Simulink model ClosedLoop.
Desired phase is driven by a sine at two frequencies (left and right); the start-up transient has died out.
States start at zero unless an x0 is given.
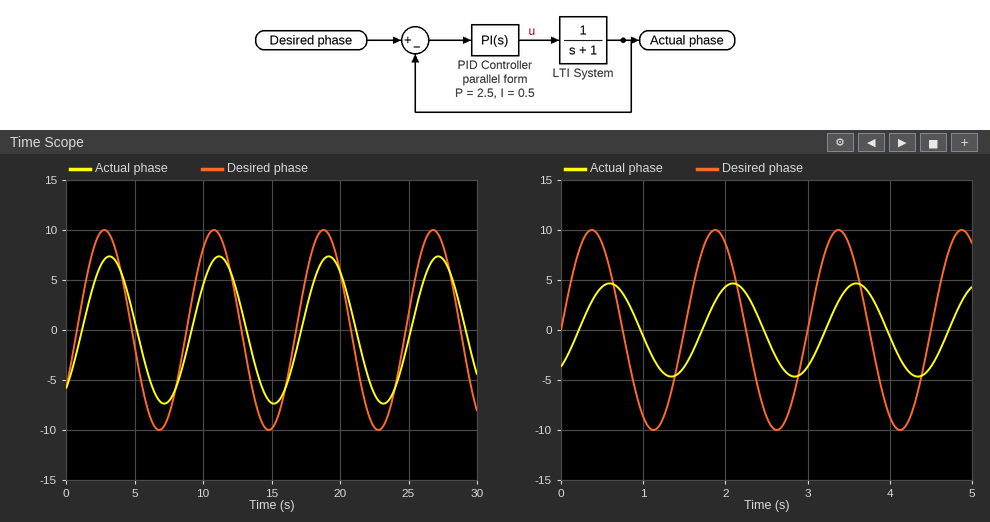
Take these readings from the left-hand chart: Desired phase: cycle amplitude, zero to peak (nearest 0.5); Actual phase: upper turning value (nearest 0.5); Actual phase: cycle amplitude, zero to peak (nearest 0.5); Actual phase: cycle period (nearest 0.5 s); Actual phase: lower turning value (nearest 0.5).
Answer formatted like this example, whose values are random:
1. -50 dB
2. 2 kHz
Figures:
1. 10.0
2. 7.5
3. 7.5
4. 8.0 s
5. -7.5
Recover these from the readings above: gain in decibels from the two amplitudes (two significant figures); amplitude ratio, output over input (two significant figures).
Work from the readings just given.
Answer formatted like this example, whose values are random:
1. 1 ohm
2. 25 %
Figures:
1. -2.5 dB
2. 0.75
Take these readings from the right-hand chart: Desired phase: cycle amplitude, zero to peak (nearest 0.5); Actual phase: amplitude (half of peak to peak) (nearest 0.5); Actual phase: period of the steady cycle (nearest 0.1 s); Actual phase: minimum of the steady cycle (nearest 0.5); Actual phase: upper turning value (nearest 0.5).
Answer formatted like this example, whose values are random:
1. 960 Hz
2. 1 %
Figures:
1. 10.0
2. 4.5
3. 1.5 s
4. -4.5
5. 4.5
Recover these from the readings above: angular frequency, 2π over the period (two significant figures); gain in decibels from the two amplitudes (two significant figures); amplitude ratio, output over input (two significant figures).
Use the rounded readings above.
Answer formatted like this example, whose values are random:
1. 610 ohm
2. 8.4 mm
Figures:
1. 4.2 rad/s
2. -6.9 dB
3. 0.45
